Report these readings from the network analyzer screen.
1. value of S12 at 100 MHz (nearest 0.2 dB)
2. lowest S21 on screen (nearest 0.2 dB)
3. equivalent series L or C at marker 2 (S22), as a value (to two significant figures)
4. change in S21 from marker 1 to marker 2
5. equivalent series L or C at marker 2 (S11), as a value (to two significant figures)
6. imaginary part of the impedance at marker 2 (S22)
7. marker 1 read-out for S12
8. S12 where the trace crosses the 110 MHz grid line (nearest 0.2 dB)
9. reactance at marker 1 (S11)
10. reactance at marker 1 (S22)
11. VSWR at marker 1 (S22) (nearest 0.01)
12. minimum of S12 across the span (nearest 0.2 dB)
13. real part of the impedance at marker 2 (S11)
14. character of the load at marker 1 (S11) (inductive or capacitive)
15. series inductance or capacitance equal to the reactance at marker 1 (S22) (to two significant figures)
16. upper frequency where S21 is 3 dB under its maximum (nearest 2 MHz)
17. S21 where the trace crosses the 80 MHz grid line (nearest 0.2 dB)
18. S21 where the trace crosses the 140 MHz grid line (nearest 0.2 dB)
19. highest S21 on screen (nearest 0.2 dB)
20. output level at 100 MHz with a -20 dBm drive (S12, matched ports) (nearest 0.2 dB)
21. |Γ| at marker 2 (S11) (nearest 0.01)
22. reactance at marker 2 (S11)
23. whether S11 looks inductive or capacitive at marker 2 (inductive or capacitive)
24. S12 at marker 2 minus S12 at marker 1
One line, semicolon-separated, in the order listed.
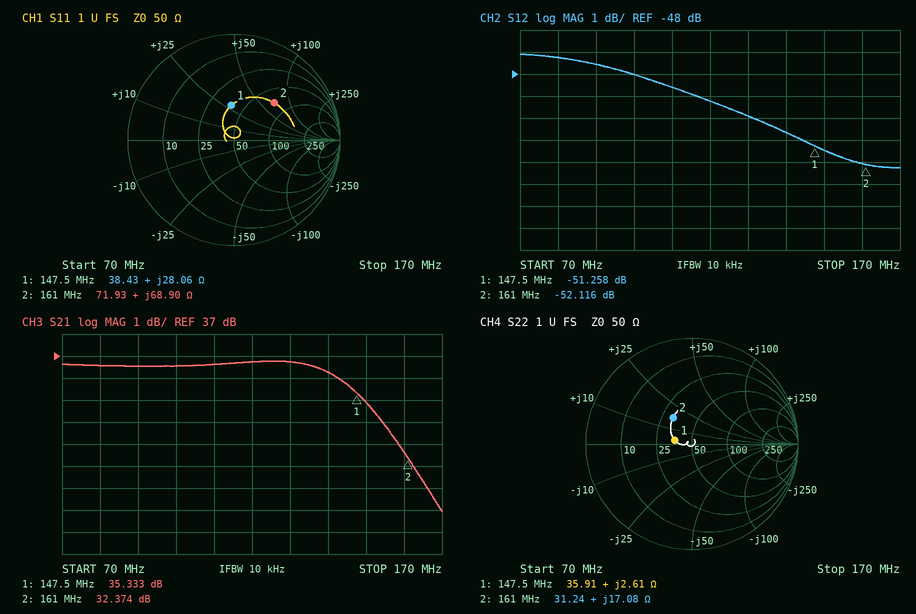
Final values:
-48.0 dB; 30.0 dB; 17 nH; -2.959 dB; 68 nH; +17.08 Ω; -51.258 dB; -48.6 dB; +28.06 Ω; +2.61 Ω; 1.40; -52.2 dB; 71.93 Ω; inductive; 2.8 nH; 156 MHz; 36.6 dB; 36.2 dB; 36.8 dB; -68.0 dBm; 0.52; +68.90 Ω; inductive; -0.858 dB
